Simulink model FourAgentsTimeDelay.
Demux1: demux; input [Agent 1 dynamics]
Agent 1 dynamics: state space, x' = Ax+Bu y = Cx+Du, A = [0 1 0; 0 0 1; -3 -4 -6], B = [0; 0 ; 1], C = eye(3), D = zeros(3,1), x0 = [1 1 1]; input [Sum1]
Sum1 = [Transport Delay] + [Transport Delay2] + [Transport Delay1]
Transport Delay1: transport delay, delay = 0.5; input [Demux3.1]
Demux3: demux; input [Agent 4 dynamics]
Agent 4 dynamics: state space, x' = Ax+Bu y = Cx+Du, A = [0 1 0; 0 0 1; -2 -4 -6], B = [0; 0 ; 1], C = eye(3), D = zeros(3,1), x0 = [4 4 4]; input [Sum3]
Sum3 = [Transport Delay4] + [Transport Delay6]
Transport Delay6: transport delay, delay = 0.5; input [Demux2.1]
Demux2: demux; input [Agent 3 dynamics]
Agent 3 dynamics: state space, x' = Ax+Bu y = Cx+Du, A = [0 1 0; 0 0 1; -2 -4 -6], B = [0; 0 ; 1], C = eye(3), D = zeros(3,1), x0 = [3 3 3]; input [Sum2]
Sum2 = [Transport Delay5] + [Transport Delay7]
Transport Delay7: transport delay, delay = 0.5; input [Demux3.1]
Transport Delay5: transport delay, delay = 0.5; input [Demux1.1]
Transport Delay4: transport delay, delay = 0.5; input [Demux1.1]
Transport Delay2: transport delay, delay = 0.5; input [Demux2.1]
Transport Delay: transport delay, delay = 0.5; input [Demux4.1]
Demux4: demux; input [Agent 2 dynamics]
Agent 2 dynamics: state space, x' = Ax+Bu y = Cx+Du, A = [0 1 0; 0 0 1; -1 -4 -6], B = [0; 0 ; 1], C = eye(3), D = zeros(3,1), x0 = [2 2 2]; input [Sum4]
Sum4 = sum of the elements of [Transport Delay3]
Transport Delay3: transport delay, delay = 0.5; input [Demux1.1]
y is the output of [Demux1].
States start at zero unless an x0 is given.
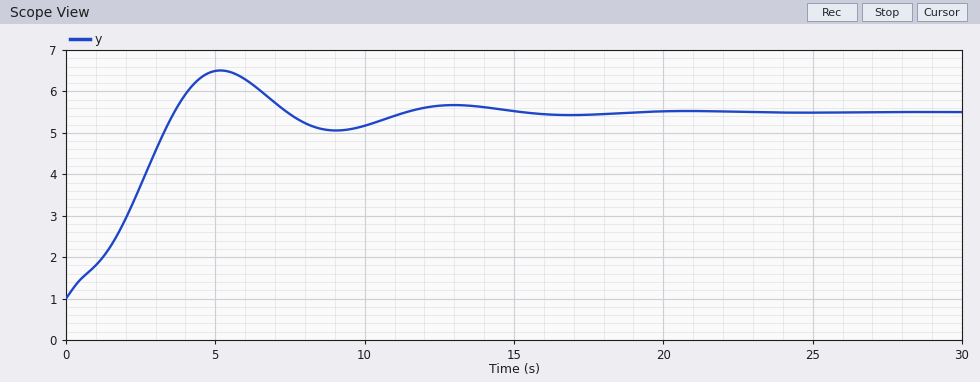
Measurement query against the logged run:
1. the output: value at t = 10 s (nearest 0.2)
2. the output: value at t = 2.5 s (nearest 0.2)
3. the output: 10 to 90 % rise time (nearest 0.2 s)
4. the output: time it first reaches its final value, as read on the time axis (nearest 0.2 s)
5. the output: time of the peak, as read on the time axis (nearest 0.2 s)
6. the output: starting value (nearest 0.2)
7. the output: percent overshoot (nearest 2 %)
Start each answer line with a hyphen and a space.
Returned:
- 5.2
- 3.8
- 2.8 s
- 3.6 s
- 5.2 s
- 1.0
- 22 %
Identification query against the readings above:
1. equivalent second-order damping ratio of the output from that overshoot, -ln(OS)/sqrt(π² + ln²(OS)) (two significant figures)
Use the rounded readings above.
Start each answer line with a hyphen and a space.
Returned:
- 0.43
